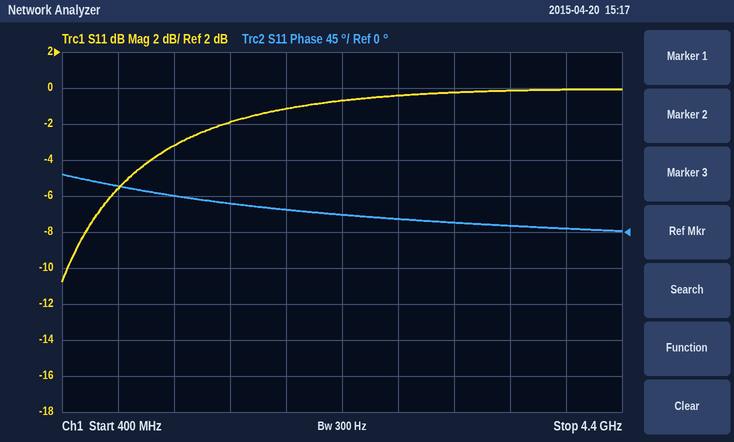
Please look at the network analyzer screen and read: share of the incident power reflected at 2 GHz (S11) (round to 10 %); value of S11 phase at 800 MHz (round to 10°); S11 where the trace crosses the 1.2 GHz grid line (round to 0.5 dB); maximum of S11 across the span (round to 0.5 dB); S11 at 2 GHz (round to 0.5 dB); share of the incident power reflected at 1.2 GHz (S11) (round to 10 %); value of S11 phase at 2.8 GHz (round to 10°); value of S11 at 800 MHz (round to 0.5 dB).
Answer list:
80 %
60°
-3.0 dB
0.0 dB
-1.0 dB
50 %
20°
-5.5 dB
